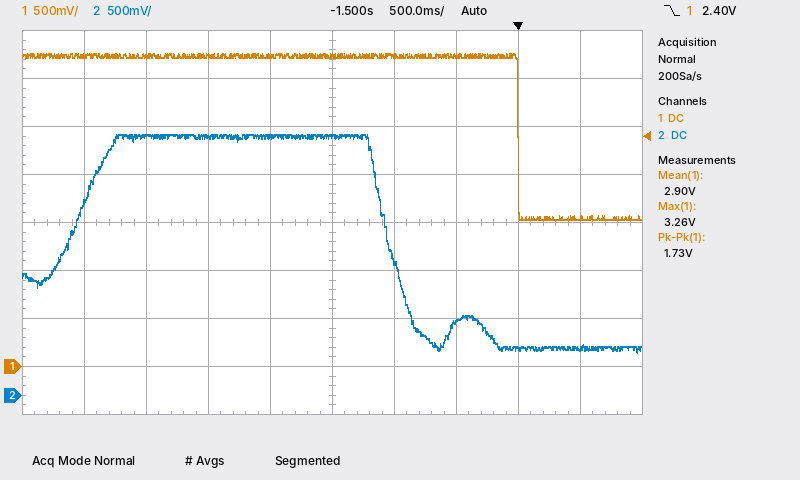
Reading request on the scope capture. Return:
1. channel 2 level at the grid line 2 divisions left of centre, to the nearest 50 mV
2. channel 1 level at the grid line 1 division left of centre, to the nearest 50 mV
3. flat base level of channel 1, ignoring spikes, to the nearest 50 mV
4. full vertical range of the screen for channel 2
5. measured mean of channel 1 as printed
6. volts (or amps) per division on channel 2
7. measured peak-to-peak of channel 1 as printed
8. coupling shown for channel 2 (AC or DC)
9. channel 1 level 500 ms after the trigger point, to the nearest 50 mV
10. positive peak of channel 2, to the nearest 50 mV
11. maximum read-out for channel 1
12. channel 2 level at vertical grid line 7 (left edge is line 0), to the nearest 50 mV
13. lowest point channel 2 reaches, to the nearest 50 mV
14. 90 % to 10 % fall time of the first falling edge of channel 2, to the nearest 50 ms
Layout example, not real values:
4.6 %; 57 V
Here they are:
2.70 V; 3.25 V; 1.55 V; 4 V; 2.90 V; 500 mV; 1.73 V; DC; 1.55 V; 2.70 V; 3.26 V; 750 mV; 450 mV; 350 ms
